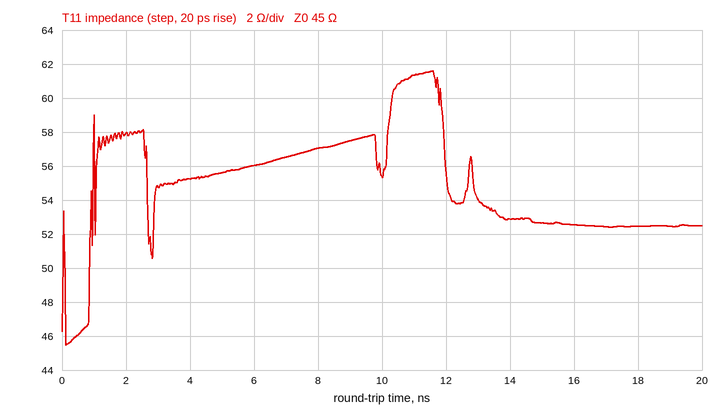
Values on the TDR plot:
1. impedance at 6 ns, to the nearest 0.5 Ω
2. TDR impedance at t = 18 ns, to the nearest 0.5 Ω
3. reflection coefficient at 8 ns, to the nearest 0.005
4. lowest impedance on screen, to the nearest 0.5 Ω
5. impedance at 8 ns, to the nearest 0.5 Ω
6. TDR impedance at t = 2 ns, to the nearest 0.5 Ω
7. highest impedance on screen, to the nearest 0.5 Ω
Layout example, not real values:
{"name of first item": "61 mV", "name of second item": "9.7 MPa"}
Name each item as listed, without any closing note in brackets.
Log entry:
{"impedance at 6 ns, to the nearest 0.5 Ω": "56.0 Ω", "TDR impedance at t = 18 ns, to the nearest 0.5 Ω": "52.5 Ω", "reflection coefficient at 8 ns, to the nearest 0.005": "+0.120", "lowest impedance on screen, to the nearest 0.5 Ω": "45.5 Ω", "impedance at 8 ns, to the nearest 0.5 Ω": "57.0 Ω", "TDR impedance at t = 2 ns, to the nearest 0.5 Ω": "58.0 Ω", "highest impedance on screen, to the nearest 0.5 Ω": "61.5 Ω"}
